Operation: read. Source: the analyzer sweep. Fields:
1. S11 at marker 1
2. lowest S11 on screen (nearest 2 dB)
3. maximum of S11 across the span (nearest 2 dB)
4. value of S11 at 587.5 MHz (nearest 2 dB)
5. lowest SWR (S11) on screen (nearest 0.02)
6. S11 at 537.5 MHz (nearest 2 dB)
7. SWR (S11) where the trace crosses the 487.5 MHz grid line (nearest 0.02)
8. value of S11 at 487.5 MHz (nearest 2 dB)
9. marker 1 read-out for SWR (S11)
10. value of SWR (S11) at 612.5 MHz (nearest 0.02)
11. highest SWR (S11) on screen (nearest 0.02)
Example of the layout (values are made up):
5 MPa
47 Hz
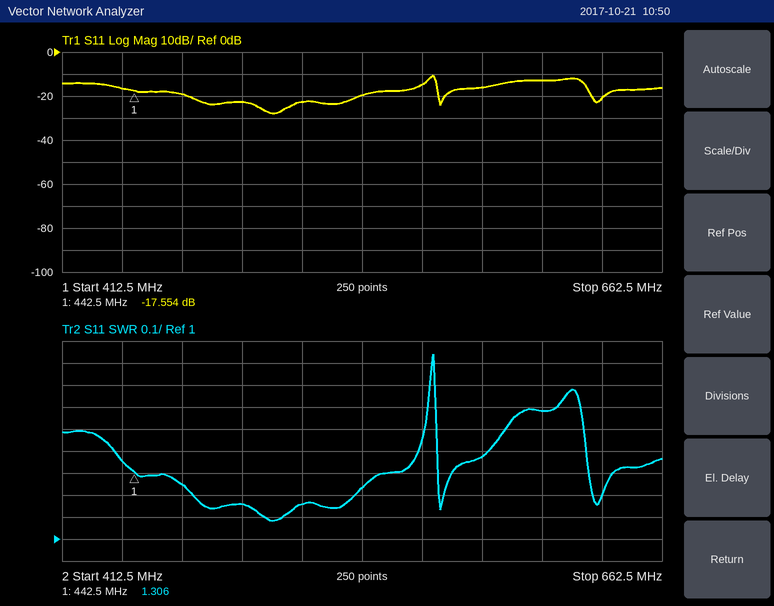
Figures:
-17.554 dB
-28 dB
-10 dB
-16 dB
1.08
-20 dB
1.16
-22 dB
1.306
1.58
1.84
